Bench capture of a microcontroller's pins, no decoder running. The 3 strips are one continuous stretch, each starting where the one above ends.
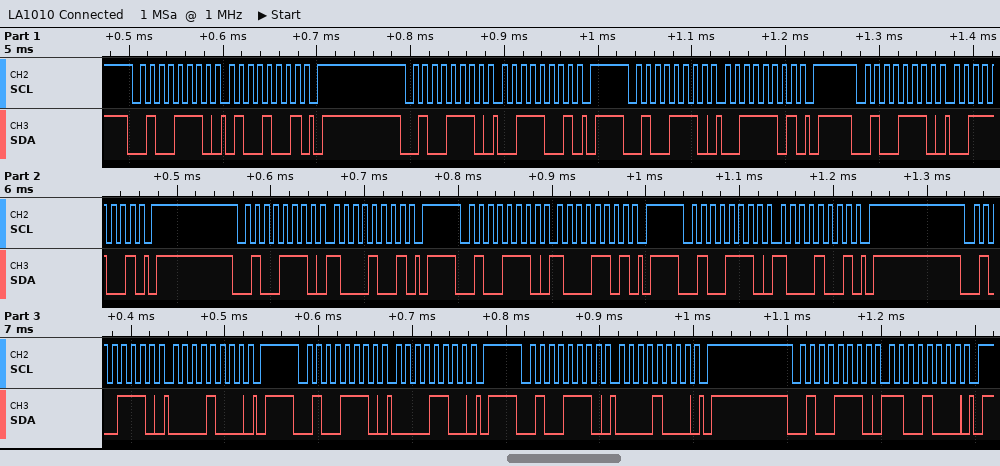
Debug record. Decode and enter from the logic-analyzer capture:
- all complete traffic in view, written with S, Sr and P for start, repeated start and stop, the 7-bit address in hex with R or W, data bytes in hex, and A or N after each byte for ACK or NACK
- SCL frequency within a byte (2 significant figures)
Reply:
S 27W A 49 A P S 27W A 39 A P S 27W A 3D A P S 27W A 39 A P S 27W A 89 A P S 27W A 8D A P S 27W A 89 A P S 27W A 08 A P S 27W A 0C A P S 27W A 08 A P S 27W A C8 A P
100 kHz
